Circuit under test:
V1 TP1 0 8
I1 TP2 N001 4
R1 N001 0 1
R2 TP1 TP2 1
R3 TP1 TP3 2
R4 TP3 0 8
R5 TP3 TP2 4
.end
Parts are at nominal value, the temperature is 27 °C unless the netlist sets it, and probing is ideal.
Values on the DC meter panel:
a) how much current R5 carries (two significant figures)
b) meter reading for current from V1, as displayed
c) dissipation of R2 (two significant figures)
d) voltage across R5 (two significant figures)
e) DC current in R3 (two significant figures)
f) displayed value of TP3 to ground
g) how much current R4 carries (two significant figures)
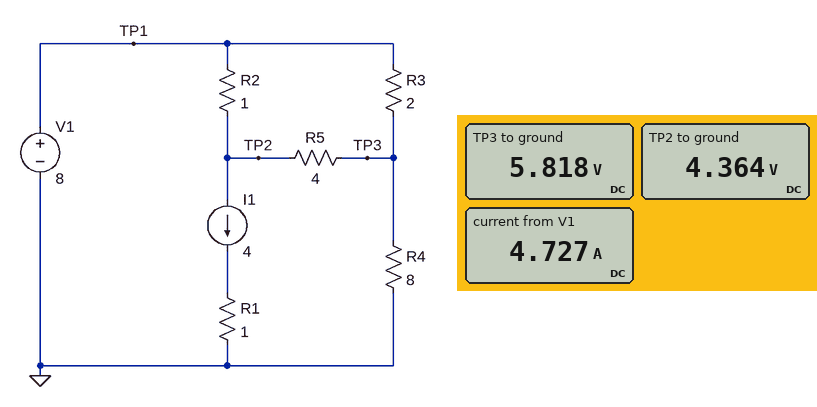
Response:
360 mA
4.727 A
13 W
1.5 V
1.1 A
5.818 V
730 mA
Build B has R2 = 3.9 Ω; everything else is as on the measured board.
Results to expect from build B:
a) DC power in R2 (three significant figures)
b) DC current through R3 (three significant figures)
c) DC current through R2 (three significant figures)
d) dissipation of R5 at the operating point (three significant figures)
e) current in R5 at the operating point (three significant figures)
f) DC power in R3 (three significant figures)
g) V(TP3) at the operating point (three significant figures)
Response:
24.9 W
1.98 A
2.53 A
8.69 W
1.47 A
7.83 W
4.04 V
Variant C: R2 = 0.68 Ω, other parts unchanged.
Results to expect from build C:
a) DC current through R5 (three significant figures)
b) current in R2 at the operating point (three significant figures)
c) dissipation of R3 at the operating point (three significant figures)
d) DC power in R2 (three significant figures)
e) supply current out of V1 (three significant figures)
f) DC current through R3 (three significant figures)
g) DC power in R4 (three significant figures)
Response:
178 mA
3.82 A
1.78 W
9.93 W
4.76 A
943 mA
4.67 W
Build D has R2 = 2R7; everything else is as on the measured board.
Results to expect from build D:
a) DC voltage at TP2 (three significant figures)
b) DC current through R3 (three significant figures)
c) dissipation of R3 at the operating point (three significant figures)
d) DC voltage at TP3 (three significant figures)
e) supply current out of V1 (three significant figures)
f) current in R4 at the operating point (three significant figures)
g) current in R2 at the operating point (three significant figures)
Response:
193 mV
1.69 A
5.69 W
4.63 V
4.58 A
578 mA
2.89 A
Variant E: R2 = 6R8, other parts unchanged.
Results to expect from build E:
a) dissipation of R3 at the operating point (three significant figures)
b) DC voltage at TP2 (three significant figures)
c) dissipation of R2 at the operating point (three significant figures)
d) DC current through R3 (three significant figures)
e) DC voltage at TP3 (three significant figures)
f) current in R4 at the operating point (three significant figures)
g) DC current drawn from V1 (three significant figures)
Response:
12.0 W
-5.16 V
25.5 W
2.45 A
3.10 V
387 mA
4.39 A
